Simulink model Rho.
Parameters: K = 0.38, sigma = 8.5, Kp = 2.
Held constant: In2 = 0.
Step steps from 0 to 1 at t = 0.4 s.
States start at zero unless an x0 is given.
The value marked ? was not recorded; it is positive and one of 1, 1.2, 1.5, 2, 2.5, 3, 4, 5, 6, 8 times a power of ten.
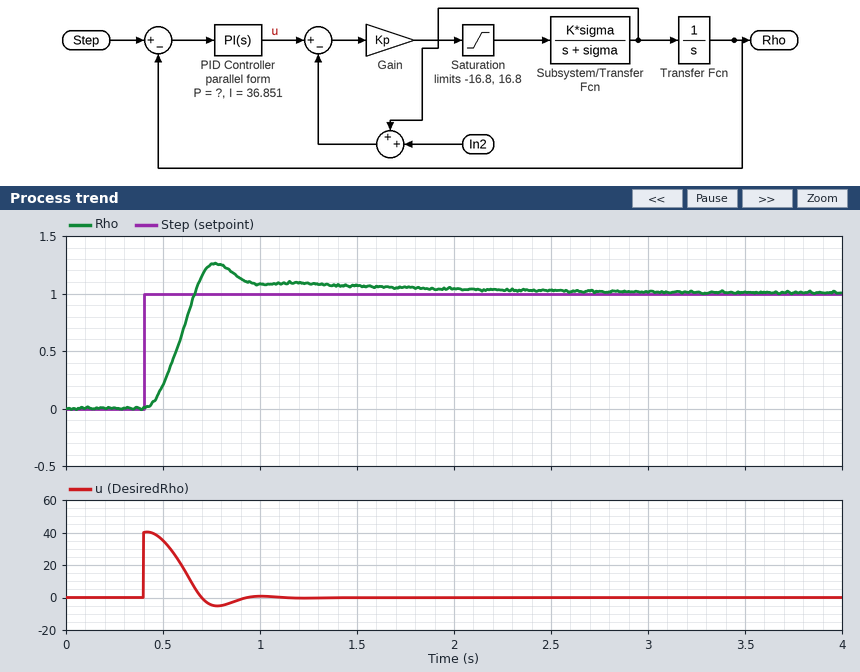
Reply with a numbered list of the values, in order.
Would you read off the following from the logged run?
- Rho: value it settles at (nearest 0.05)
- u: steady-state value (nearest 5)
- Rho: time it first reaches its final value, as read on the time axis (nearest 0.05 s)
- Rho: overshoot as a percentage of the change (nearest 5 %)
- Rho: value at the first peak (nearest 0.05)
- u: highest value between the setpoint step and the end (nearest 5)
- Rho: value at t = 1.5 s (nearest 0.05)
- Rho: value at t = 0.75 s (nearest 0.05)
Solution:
1. 1.00
2. 0
3. 0.65 s
4. 25 %
5. 1.25
6. 40
7. 1.05
8. 1.25
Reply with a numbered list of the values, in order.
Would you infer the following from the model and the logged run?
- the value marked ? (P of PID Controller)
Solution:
1. 40
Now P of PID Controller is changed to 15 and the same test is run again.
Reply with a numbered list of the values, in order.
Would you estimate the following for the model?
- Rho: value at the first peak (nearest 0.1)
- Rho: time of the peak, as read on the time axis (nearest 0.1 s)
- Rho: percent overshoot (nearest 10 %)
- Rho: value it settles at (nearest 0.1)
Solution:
1. 1.4
2. 0.9 s
3. 40 %
4. 1.0
